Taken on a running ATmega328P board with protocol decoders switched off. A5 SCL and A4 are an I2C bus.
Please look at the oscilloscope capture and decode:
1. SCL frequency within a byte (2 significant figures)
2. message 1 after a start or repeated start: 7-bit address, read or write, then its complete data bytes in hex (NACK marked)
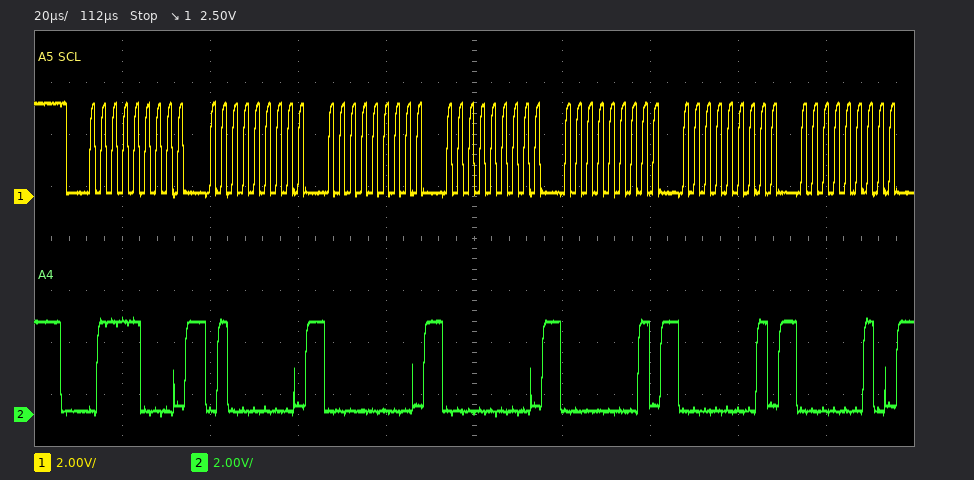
400 kHz
0x3C write: 40 00 00 01 01 02
